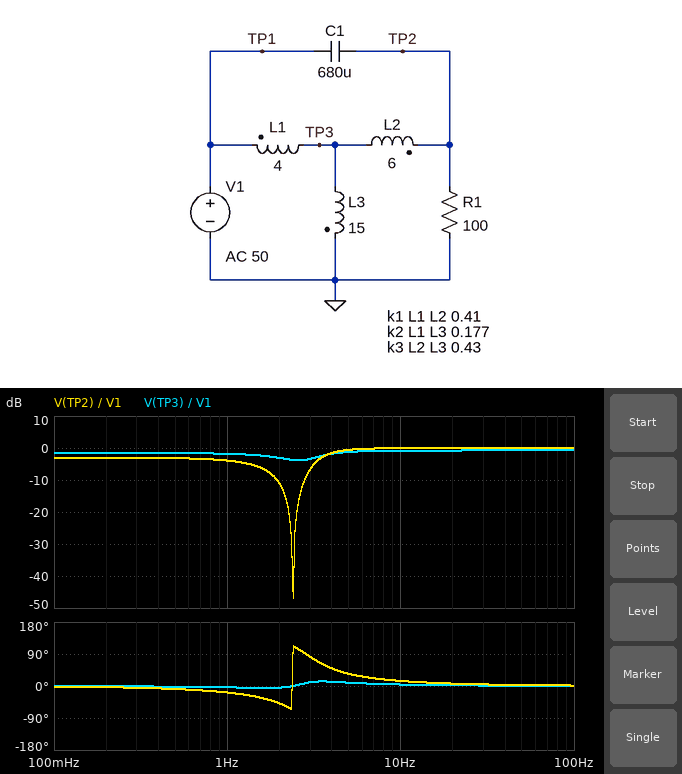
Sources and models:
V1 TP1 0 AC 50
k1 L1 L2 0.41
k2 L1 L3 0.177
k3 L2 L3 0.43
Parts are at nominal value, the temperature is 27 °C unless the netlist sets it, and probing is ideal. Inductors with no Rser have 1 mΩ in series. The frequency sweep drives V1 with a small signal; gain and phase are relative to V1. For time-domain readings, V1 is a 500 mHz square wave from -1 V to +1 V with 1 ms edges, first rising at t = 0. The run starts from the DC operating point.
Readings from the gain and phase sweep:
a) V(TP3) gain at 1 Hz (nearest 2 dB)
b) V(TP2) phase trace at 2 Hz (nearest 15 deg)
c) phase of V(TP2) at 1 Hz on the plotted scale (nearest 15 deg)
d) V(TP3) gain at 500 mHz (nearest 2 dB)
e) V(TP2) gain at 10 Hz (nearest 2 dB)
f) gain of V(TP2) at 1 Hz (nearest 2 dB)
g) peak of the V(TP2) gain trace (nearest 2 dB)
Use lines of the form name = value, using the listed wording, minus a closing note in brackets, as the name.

V(TP3) gain at 1 Hz = -2 dB
V(TP2) phase trace at 2 Hz = -45 deg
phase of V(TP2) at 1 Hz on the plotted scale = -15 deg
V(TP3) gain at 500 mHz = -2 dB
V(TP2) gain at 10 Hz = 0 dB
gain of V(TP2) at 1 Hz = -4 dB
peak of the V(TP2) gain trace = 0 dB
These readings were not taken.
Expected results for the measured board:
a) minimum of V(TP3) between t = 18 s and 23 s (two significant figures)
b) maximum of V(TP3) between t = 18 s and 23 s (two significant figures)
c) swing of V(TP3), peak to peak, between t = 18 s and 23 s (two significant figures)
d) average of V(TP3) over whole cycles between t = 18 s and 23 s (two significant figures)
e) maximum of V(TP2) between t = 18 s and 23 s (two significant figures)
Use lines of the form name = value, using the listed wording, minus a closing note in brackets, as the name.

minimum of V(TP3) between t = 18 s and 23 s = -650 mV
maximum of V(TP3) between t = 18 s and 23 s = 1.3 V
swing of V(TP3), peak to peak, between t = 18 s and 23 s = 2.0 V
average of V(TP3) over whole cycles between t = 18 s and 23 s = 340 mV
maximum of V(TP2) between t = 18 s and 23 s = 1.5 V
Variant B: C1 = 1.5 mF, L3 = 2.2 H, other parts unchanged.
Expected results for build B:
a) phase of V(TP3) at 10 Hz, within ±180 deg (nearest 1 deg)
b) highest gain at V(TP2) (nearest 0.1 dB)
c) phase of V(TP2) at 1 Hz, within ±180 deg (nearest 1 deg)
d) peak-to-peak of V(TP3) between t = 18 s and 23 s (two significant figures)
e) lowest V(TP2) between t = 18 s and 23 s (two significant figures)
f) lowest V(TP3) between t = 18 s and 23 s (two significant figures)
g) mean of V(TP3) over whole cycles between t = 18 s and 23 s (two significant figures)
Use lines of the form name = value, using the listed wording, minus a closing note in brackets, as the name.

phase of V(TP3) at 10 Hz, within ±180 deg = 0 deg
highest gain at V(TP2) = 2.5 dB
phase of V(TP2) at 1 Hz, within ±180 deg = -19 deg
peak-to-peak of V(TP3) between t = 18 s and 23 s = 670 mV
lowest V(TP2) between t = 18 s and 23 s = -1.6 V
lowest V(TP3) between t = 18 s and 23 s = -510 mV
mean of V(TP3) over whole cycles between t = 18 s and 23 s = -170 mV
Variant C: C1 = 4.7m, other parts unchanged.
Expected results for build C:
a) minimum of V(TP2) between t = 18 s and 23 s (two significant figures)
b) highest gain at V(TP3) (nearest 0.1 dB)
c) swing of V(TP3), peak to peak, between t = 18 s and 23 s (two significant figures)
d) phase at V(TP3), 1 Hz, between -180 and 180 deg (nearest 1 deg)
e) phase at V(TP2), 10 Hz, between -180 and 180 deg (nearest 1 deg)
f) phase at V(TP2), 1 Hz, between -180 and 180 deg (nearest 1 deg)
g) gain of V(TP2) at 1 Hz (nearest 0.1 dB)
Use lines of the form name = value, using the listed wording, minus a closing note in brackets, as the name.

minimum of V(TP2) between t = 18 s and 23 s = -980 mV
highest gain at V(TP3) = -0.5 dB
swing of V(TP3), peak to peak, between t = 18 s and 23 s = 1.9 V
phase at V(TP3), 1 Hz, between -180 and 180 deg = 10 deg
phase at V(TP2), 10 Hz, between -180 and 180 deg = 2 deg
phase at V(TP2), 1 Hz, between -180 and 180 deg = 116 deg
gain of V(TP2) at 1 Hz = -6.8 dB
